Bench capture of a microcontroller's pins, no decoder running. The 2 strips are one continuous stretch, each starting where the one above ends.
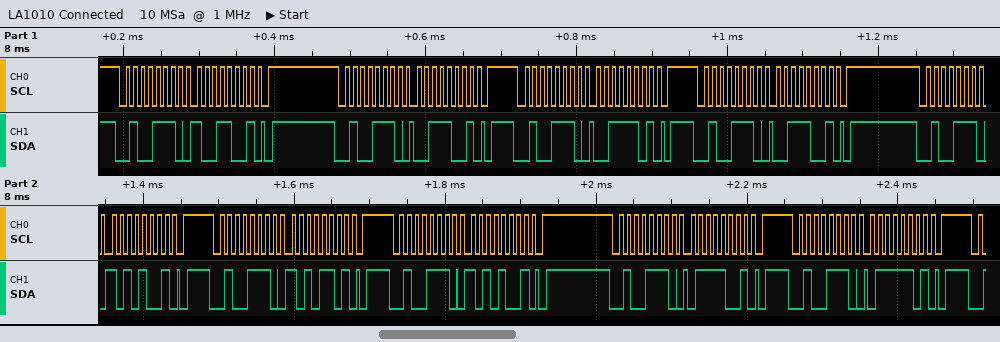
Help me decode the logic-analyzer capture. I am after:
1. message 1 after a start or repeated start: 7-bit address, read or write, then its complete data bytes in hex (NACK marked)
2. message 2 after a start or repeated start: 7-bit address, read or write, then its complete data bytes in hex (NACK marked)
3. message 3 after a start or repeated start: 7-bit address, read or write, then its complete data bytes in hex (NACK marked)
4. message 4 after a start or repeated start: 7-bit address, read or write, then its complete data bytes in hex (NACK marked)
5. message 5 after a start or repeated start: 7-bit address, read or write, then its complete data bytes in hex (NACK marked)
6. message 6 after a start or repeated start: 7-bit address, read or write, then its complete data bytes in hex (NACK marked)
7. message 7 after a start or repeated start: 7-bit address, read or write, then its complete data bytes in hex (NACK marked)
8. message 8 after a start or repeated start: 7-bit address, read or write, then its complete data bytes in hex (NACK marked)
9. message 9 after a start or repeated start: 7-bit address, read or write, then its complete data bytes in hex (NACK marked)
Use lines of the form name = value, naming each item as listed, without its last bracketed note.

message 1 after a start or repeated start: 7-bit address, read or write, then its complete data bytes in hex = 0x27 write: 99
message 2 after a start or repeated start: 7-bit address, read or write, then its complete data bytes in hex = 0x27 write: 39
message 3 after a start or repeated start: 7-bit address, read or write, then its complete data bytes in hex = 0x27 write: 3D
message 4 after a start or repeated start: 7-bit address, read or write, then its complete data bytes in hex = 0x27 write: 39
message 5 after a start or repeated start: 7-bit address, read or write, then its complete data bytes in hex = 0x27 write: A9
message 6 after a start or repeated start: 7-bit address, read or write, then its complete data bytes in hex = 0x27 write: AD
message 7 after a start or repeated start: 7-bit address, read or write, then its complete data bytes in hex = 0x27 write: A9
message 8 after a start or repeated start: 7-bit address, read or write, then its complete data bytes in hex = 0x27 write: 79
message 9 after a start or repeated start: 7-bit address, read or write, then its complete data bytes in hex = 0x27 write: 7D
